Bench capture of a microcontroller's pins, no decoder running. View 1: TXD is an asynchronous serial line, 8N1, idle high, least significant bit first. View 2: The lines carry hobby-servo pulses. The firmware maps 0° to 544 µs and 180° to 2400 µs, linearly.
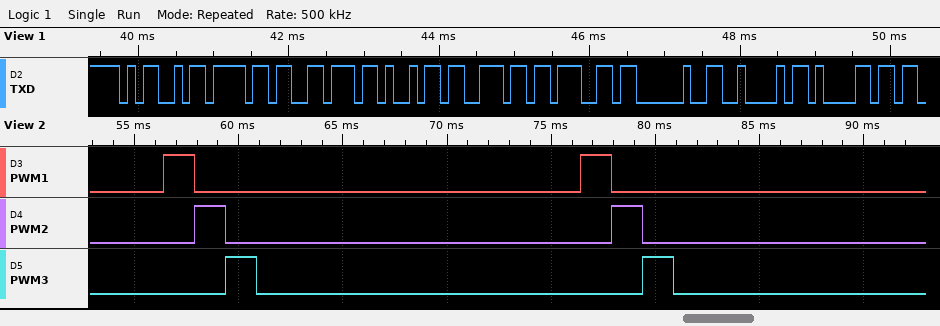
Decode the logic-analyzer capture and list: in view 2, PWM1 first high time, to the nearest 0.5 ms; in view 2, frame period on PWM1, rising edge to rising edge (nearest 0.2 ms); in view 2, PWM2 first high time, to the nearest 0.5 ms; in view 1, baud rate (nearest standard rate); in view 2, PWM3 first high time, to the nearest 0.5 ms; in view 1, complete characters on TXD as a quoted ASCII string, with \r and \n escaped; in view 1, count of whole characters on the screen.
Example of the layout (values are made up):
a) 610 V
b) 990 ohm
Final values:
a) 1.5 ms
b) 20.0 ms
c) 1.5 ms
d) 9600 baud
e) 1.5 ms
f) "Moving Ba"
g) 9
